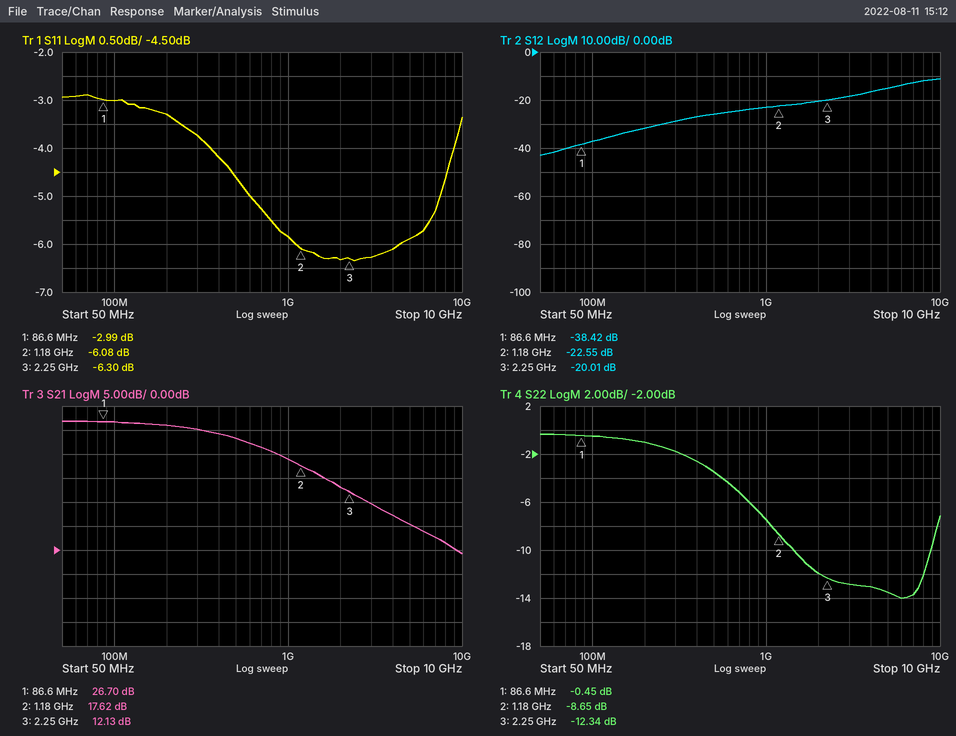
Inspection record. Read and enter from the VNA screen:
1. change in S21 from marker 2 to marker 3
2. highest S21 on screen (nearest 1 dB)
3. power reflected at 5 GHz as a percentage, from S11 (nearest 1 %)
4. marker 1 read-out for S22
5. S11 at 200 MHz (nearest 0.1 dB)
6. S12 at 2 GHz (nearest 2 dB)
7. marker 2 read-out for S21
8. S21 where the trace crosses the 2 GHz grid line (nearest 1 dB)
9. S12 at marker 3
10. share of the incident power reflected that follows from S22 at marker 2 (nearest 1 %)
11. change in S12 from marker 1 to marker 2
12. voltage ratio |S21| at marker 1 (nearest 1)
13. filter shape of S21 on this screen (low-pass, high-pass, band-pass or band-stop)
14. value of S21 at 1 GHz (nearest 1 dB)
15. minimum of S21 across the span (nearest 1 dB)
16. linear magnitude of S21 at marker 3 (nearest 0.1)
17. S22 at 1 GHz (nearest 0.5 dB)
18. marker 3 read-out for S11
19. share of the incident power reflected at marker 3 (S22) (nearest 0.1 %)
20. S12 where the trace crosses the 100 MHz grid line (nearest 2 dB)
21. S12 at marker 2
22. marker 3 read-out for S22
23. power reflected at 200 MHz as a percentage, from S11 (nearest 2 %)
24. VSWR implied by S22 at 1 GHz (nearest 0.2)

-5.49 dB
27 dB
26 %
-0.45 dB
-3.3 dB
-20 dB
17.62 dB
13 dB
-20.01 dB
14 %
15.87 dB
22
low-pass
19 dB
-1 dB
4.0
-7.5 dB
-6.30 dB
5.8 %
-38 dB
-22.55 dB
-12.34 dB
46 %
2.4
